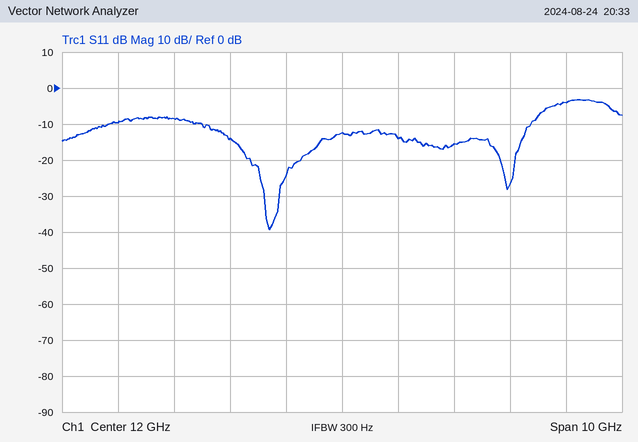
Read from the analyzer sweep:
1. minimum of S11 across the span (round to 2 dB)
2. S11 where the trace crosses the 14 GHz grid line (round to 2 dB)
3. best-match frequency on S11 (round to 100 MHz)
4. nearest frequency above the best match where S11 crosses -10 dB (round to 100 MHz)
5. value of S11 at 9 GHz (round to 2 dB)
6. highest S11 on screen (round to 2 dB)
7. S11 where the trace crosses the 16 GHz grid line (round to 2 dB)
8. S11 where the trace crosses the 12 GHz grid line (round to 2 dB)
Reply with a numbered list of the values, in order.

1. -40 dB
2. -16 dB
3. 10.7 GHz
4. 15.4 GHz
5. -8 dB
6. -4 dB
7. -4 dB
8. -12 dB
